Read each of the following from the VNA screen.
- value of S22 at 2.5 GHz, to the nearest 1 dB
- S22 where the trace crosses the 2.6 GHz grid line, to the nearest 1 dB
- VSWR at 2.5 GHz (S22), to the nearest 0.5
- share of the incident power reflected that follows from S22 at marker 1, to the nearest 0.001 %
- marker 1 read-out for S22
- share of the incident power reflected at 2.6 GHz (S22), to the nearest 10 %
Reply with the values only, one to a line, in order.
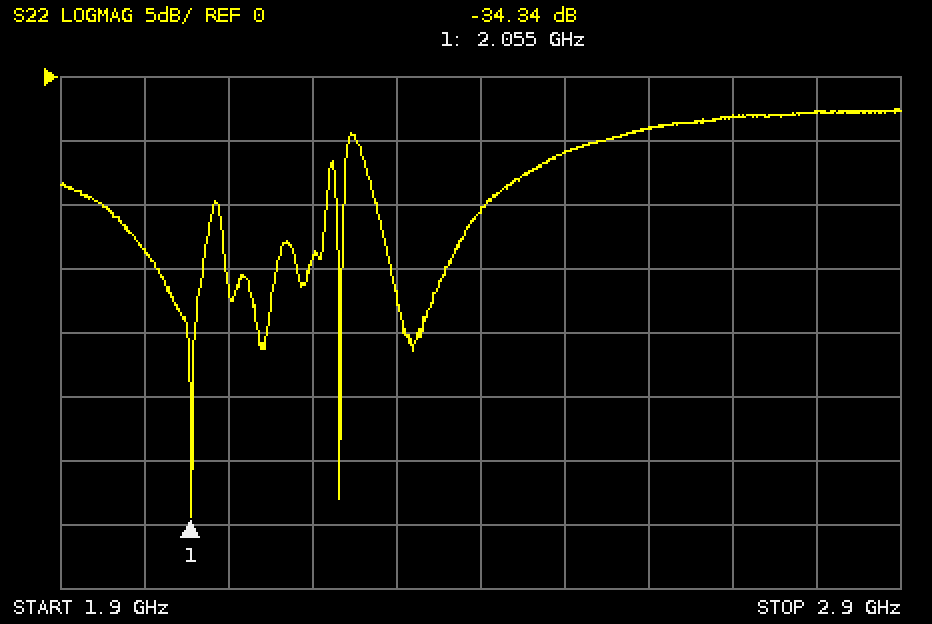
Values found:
-6 dB
-4 dB
3.0
0.037 %
-34.34 dB
40 %
